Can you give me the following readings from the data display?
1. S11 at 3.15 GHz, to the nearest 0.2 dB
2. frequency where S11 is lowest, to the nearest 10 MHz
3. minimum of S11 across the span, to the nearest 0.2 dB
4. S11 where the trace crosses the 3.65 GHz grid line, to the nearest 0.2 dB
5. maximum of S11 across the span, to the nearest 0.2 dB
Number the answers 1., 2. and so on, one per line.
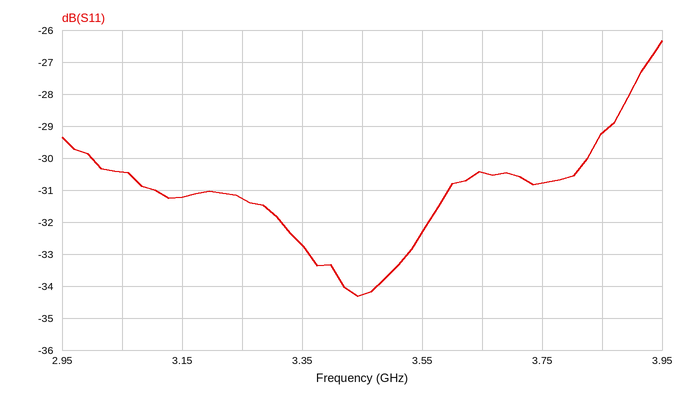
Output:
1. -31.2 dB
2. 3.44 GHz
3. -34.4 dB
4. -30.4 dB
5. -26.4 dB
